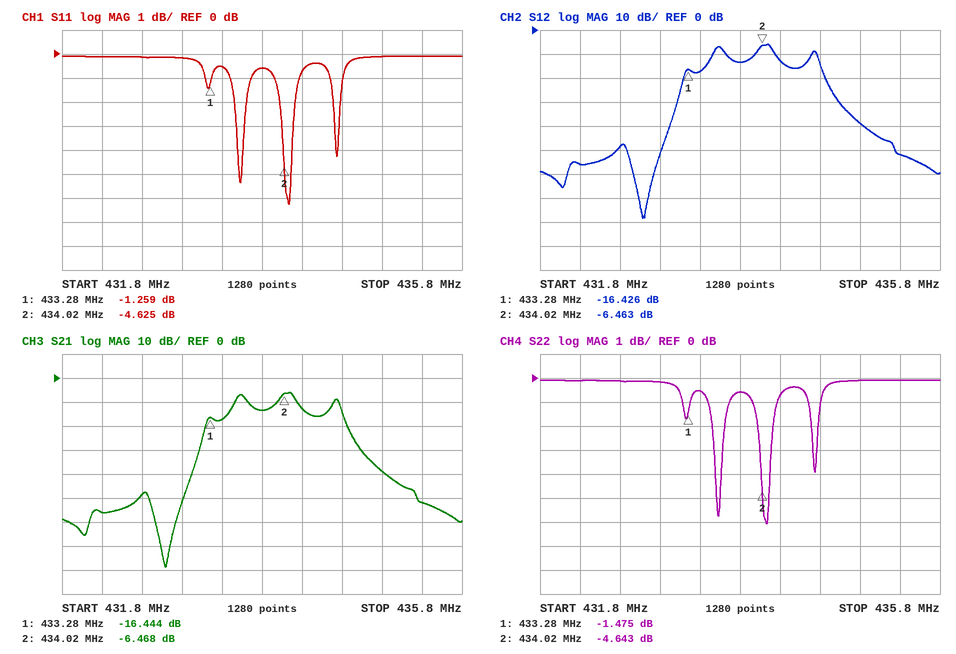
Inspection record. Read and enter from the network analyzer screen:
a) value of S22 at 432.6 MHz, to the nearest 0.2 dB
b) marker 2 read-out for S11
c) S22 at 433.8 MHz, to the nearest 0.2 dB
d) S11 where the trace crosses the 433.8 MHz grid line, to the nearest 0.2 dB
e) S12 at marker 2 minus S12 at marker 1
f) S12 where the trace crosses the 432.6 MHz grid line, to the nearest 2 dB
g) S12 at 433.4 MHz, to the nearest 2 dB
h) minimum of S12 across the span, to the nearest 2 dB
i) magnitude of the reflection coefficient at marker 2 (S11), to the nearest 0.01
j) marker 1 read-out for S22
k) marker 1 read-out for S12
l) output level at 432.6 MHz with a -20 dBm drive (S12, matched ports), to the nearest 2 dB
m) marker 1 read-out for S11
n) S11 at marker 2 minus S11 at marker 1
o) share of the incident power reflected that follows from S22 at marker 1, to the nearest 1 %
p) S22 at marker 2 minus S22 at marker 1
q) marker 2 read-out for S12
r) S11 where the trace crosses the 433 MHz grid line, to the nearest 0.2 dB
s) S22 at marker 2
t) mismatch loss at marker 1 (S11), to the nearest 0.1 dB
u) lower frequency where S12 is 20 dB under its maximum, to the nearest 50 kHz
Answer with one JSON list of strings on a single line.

["-0.2 dB", "-4.625 dB", "-0.6 dB", "-0.6 dB", "9.963 dB", "-48 dB", "-18 dB", "-78 dB", "0.59", "-1.475 dB", "-16.426 dB", "-68 dBm", "-1.259 dB", "-3.366 dB", "71 %", "-3.168 dB", "-6.463 dB", "-0.2 dB", "-4.643 dB", "6.0 dB", "433.20 MHz"]
